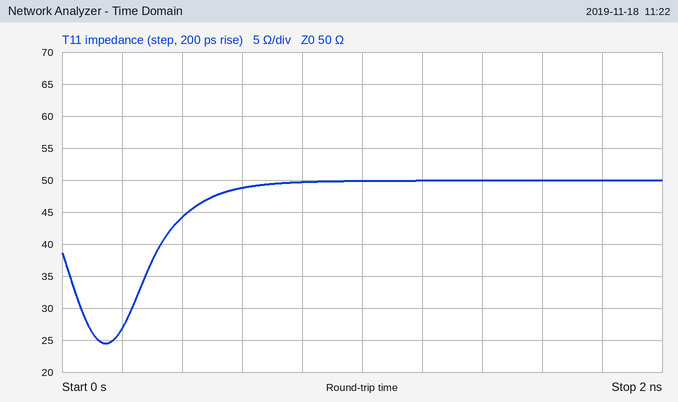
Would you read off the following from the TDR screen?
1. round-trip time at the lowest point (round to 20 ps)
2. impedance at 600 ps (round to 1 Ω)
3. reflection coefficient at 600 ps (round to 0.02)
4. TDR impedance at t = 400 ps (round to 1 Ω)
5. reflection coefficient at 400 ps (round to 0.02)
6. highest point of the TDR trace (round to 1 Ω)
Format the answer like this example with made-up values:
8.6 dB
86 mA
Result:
140 ps
49 Ω
-0.02
44 Ω
-0.06
50 Ω
